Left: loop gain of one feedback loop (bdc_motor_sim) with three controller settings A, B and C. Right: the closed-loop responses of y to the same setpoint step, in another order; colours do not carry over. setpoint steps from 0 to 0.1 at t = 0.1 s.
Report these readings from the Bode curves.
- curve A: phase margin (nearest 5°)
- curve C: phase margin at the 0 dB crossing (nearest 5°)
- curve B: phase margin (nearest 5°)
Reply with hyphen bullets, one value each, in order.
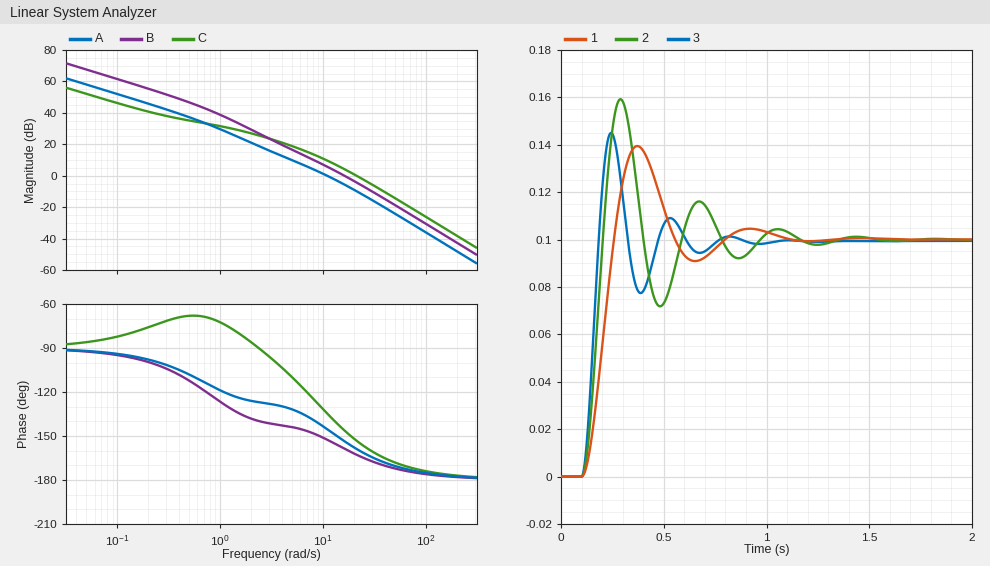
- 35°
- 25°
- 20°
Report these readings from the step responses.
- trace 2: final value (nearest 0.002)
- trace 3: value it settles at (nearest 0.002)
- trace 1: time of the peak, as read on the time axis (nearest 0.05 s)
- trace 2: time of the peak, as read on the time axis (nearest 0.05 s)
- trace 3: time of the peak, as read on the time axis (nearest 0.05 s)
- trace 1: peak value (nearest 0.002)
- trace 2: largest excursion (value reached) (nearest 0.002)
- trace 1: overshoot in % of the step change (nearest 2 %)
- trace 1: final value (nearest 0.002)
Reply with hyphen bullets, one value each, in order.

- 0.100
- 0.100
- 0.35 s
- 0.30 s
- 0.25 s
- 0.140
- 0.160
- 40 %
- 0.100
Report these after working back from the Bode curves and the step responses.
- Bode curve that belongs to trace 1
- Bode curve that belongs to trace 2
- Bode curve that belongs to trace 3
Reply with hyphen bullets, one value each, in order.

- A
- B
- C
